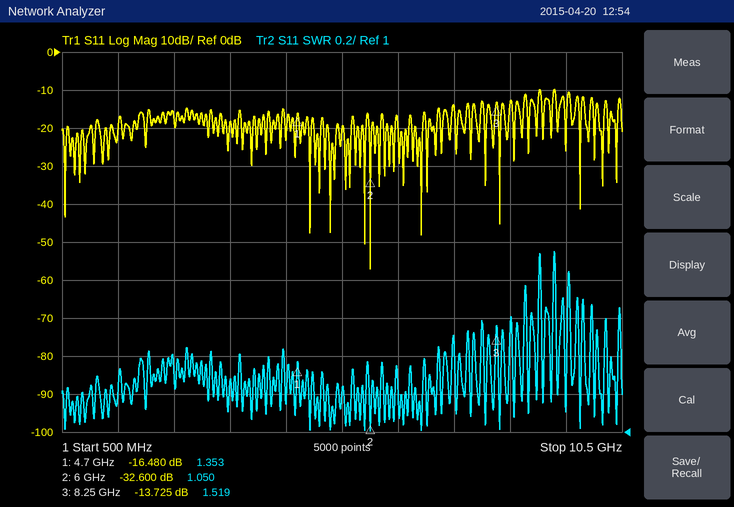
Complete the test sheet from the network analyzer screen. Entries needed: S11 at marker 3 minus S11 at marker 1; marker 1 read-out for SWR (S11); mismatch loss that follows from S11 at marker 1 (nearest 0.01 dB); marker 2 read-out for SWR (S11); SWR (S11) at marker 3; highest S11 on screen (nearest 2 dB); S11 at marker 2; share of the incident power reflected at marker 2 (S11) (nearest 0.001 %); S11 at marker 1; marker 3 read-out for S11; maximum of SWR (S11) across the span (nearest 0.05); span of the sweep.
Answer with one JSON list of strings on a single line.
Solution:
["2.755 dB", "1.353", "0.10 dB", "1.050", "1.519", "-10 dB", "-32.600 dB", "0.055 %", "-16.480 dB", "-13.725 dB", "1.95", "10 GHz"]
